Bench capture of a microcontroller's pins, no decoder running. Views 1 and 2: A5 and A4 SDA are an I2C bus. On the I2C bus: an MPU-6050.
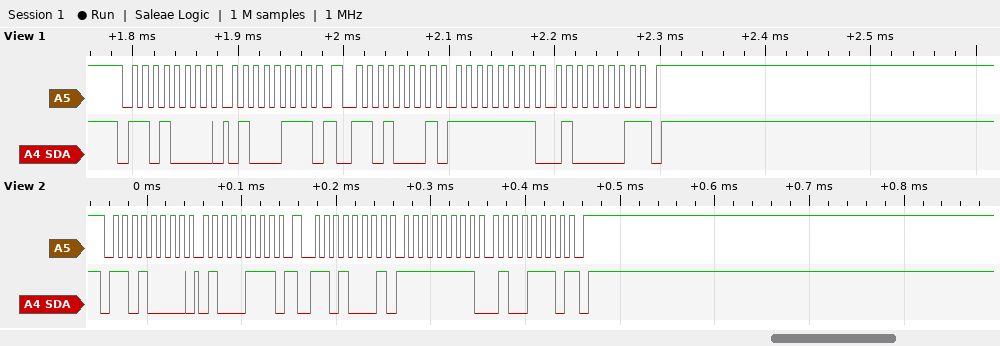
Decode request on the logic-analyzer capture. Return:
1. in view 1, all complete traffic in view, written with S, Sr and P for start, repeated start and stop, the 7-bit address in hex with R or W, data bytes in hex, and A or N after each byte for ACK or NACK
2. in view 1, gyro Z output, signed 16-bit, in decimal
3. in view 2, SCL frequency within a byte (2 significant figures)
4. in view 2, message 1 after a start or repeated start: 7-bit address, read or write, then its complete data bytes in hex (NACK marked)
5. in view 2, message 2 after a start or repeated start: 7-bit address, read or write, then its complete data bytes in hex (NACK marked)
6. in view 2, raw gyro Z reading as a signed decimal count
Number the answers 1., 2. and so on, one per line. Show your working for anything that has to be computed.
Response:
1. S 68W A 47 A Sr 68R A FF A 41 N P
2. 0xFF41 = -191
3. 100 kHz
4. 0x68 write: 47
5. 0x68 read: FF 4E NACK
6. 0xFF4E = -178
